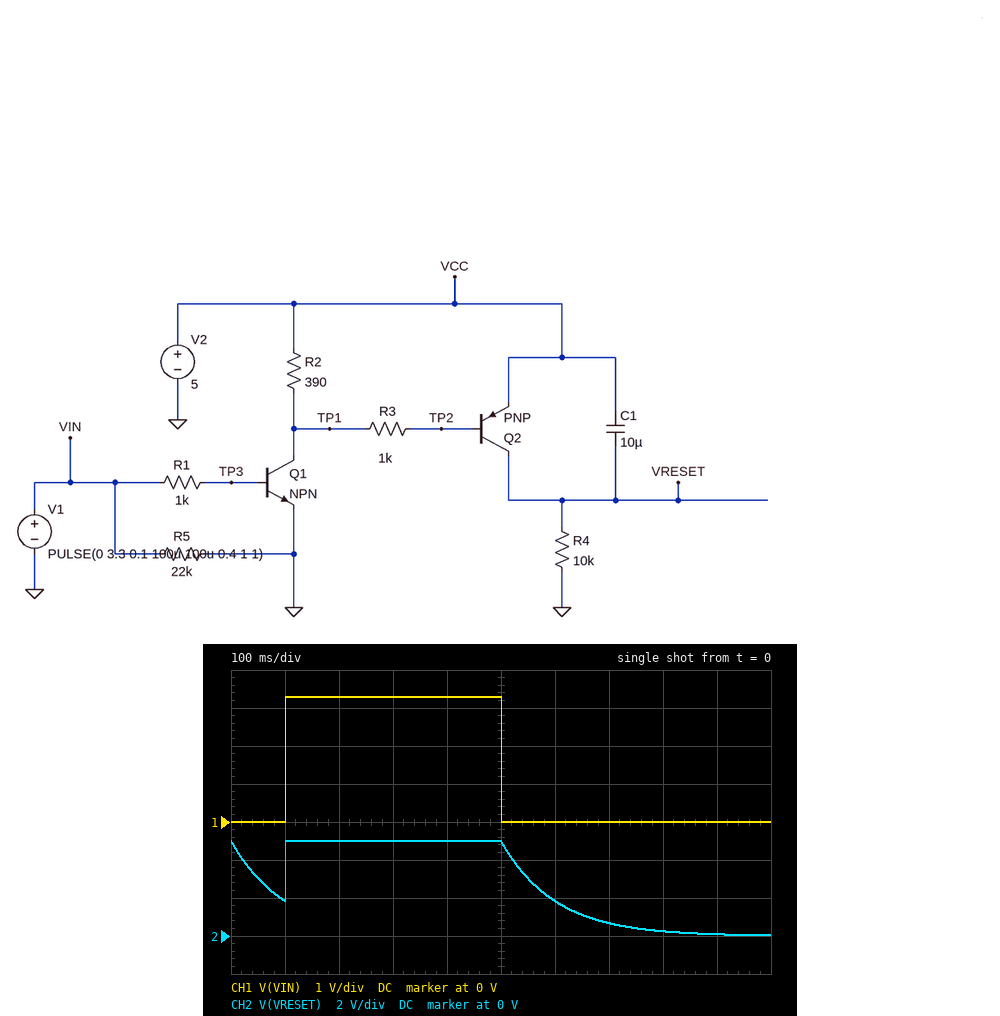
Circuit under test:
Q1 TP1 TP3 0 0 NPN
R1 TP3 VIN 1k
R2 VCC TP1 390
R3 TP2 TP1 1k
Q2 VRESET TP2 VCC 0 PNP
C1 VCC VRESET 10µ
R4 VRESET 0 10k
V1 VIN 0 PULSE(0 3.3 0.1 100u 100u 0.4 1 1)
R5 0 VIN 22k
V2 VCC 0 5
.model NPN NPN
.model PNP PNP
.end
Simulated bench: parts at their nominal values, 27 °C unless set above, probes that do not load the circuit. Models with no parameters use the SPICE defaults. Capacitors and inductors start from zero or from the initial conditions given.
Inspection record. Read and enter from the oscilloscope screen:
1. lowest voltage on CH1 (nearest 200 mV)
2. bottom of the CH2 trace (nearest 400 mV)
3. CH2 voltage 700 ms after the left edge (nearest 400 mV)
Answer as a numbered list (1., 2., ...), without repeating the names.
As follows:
1. 0 V
2. 0 V
3. 800 mV
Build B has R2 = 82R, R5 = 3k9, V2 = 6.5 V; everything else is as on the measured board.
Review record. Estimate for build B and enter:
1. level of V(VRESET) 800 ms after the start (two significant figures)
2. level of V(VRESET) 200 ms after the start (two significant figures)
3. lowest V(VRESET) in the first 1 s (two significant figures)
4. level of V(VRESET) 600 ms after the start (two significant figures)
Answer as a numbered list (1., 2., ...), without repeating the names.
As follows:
1. 320 mV
2. 6.5 V
3. 44 mV
4. 2.4 V
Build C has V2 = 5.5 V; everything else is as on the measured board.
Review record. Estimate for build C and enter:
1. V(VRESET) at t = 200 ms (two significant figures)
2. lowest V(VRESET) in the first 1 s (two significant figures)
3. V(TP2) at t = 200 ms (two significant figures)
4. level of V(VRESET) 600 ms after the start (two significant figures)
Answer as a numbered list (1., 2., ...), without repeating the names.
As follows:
1. 5.5 V
2. 37 mV
3. 4.7 V
4. 2.0 V
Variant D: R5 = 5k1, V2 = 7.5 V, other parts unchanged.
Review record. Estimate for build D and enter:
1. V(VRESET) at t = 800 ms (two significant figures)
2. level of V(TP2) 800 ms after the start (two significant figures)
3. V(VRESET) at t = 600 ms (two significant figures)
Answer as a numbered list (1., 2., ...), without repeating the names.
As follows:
1. 370 mV
2. 7.5 V
3. 2.8 V
